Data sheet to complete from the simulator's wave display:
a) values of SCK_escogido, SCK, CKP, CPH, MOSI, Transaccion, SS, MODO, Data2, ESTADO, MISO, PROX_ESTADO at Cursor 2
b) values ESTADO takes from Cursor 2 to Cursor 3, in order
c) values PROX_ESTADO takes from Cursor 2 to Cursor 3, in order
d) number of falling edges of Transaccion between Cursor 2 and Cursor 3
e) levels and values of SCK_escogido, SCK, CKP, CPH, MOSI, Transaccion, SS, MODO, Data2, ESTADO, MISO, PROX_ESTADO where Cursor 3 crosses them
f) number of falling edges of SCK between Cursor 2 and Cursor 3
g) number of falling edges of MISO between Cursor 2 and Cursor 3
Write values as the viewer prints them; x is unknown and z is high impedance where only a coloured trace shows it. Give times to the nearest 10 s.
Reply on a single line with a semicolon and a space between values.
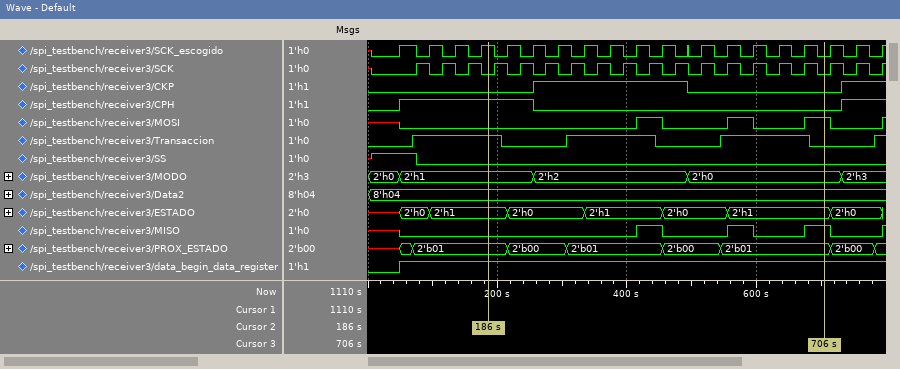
SCK_escogido=1, SCK=0, CKP=0, CPH=1, MOSI=0, Transaccion=1, SS=0, MODO=2'h1, Data2=8'h04, ESTADO=2'h1, MISO=0, PROX_ESTADO=2'b01; 2'h1, 2'h0, 2'h1, 2'h0, 2'h1; 2'b01, 2'b00, 2'b01, 2'b00, 2'b01; 3; SCK_escogido=0, SCK=0, CKP=0, CPH=0, MOSI=1, Transaccion=0, SS=0, MODO=2'h0, Data2=8'h04, ESTADO=2'h1, MISO=1, PROX_ESTADO=2'b01; 13; 2
